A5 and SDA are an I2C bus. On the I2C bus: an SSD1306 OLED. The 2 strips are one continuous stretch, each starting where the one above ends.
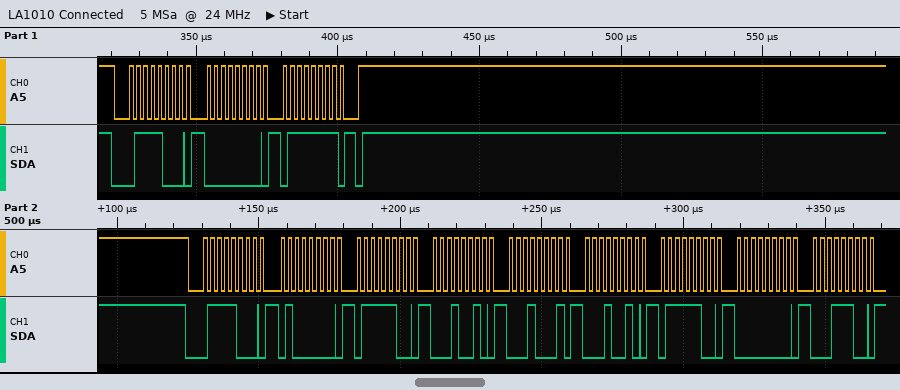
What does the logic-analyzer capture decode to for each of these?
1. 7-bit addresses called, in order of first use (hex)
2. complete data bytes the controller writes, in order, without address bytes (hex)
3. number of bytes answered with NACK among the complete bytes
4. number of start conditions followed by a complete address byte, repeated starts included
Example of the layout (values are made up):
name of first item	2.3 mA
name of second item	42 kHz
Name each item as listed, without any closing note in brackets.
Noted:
7-bit addresses called, in order of first use	0x3C
complete data bytes the controller writes, in order, without address bytes	00 7F 40 7C 12 11 12 7C 00 1C
number of bytes answered with NACK among the complete bytes	0
number of start conditions followed by a complete address byte, repeated starts included	2
